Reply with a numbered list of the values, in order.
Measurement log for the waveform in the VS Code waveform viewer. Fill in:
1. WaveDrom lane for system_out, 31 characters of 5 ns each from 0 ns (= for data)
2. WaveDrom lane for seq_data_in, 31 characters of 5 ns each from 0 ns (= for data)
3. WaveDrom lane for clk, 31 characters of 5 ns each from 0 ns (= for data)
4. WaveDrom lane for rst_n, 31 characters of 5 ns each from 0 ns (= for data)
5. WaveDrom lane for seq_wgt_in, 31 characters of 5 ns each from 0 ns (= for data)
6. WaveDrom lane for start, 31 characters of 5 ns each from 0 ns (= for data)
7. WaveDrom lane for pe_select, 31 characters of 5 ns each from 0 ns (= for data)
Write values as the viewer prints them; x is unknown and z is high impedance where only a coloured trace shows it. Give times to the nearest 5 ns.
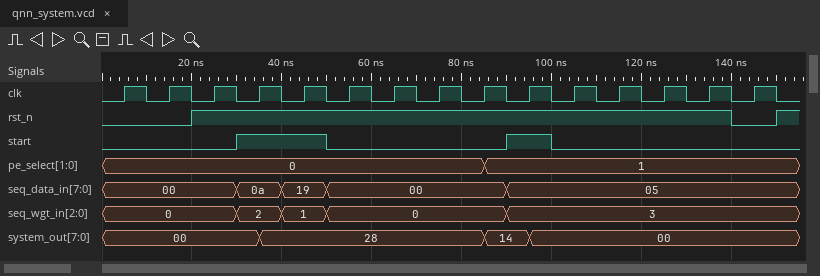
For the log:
1. {name: 'system_out', wave: '=......=.........=.=...........', data: '00 28 14 00'}
2. {name: 'seq_data_in', wave: '=.....=.=.=.......=............', data: '00 0a 19 00 05'}
3. {name: 'clk', wave: '0101010101010101010101010101010'}
4. {name: 'rst_n', wave: '0...1.......................0.1'}
5. {name: 'seq_wgt_in', wave: '=.....=.=.=.......=............', data: '0 2 1 0 3'}
6. {name: 'start', wave: '0.....1...0.......1.0..........'}
7. {name: 'pe_select', wave: '=................=.............', data: '0 1'}
